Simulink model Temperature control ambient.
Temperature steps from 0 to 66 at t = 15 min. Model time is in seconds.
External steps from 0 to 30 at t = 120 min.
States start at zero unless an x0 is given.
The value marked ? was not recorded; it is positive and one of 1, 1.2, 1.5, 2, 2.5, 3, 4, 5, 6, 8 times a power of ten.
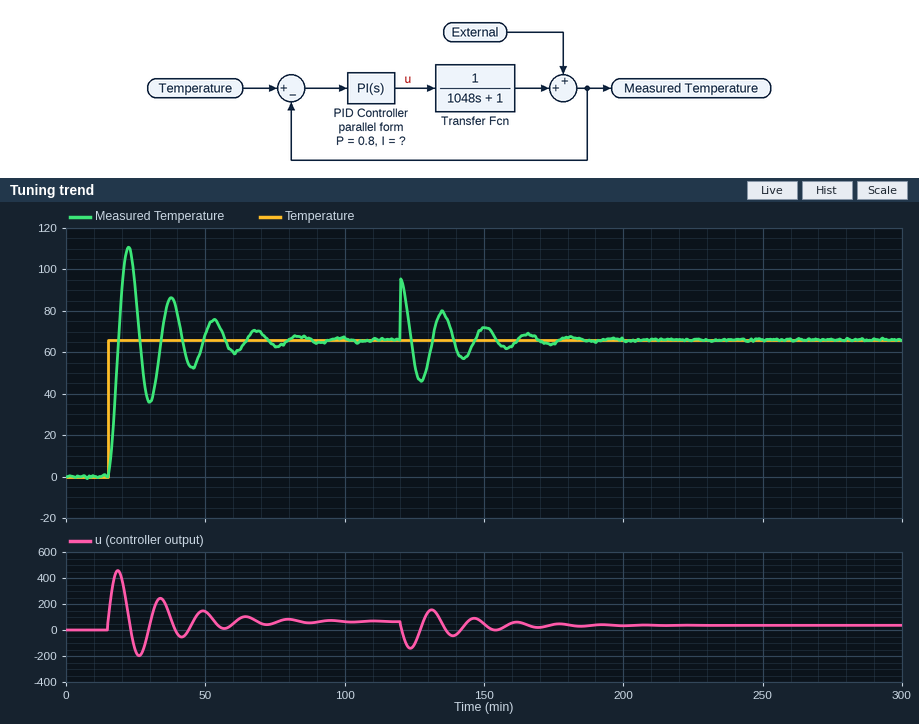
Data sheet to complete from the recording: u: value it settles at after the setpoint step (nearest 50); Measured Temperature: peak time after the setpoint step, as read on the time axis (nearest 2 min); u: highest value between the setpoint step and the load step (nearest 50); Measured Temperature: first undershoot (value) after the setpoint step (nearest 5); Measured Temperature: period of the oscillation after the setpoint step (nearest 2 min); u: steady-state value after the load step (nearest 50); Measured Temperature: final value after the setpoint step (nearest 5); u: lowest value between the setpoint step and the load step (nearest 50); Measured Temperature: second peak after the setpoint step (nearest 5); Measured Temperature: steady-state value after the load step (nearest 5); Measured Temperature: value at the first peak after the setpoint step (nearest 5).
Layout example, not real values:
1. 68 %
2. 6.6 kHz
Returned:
1. 50
2. 22 min
3. 450
4. 35
5. 16 min
6. 50
7. 65
8. -200
9. 85
10. 65
11. 110
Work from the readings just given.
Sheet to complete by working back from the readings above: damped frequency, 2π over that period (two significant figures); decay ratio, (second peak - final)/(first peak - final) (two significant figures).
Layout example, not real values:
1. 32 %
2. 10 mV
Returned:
1. 0.39 rad/min
2. 0.44
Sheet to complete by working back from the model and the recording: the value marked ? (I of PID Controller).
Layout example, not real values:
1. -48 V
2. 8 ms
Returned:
1. 0.05
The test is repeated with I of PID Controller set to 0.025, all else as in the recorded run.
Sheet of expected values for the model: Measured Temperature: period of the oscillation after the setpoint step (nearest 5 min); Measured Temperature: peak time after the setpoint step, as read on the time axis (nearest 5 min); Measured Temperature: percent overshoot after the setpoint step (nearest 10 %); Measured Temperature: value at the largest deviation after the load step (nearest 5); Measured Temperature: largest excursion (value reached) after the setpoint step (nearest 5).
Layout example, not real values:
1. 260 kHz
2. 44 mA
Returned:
1. 20 min
2. 25 min
3. 60 %
4. 95
5. 105
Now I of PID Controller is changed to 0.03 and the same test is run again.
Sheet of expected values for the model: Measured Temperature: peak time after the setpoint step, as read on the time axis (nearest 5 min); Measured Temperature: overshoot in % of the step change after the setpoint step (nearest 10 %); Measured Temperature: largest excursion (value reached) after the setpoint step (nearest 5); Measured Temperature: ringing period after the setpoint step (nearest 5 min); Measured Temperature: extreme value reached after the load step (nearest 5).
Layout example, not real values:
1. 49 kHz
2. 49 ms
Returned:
1. 25 min
2. 60 %
3. 105
4. 20 min
5. 95
